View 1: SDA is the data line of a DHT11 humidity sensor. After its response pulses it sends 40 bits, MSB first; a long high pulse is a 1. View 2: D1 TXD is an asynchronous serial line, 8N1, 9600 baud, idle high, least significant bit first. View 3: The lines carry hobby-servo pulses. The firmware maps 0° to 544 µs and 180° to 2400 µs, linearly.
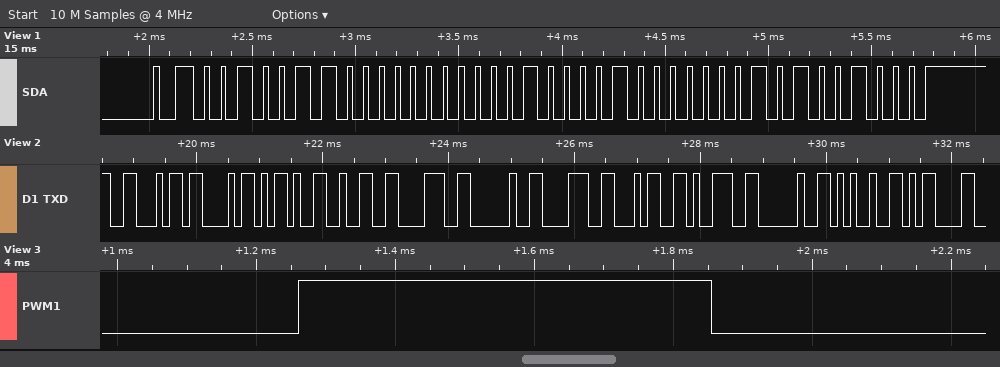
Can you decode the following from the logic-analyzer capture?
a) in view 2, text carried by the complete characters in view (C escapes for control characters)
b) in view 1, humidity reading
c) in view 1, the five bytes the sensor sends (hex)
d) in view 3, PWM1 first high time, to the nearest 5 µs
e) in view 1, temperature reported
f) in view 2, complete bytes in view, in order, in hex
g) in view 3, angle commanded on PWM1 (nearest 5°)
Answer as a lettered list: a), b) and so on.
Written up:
a) "FC-28 849 %\r"
b) 38 %
c) 26 00 21 01 48
d) 595 µs
e) 33.1 °C
f) 46 43 2D 32 38 20 38 34 39 20 25 0D
g) 5°
